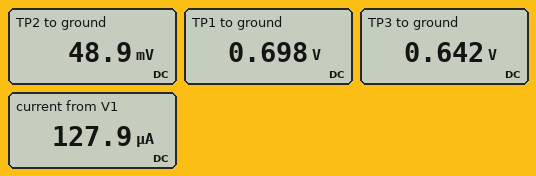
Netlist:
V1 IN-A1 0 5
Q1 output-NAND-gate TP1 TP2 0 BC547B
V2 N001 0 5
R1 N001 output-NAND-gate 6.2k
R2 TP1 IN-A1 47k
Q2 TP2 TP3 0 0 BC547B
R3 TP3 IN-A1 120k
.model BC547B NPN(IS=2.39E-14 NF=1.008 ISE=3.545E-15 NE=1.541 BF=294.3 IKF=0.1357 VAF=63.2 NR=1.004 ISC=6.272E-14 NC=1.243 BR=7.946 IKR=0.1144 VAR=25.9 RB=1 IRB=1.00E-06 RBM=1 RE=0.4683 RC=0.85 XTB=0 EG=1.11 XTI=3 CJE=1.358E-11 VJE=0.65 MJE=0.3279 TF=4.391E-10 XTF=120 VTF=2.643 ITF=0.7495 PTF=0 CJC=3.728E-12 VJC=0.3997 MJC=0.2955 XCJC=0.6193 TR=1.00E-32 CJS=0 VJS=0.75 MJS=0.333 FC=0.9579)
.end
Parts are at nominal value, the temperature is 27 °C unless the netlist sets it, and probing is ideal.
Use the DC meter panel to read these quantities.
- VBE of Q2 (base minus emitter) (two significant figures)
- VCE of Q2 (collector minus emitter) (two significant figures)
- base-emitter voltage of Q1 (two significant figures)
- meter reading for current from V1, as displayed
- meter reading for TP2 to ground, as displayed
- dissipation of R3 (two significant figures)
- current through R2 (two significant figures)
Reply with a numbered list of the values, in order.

1. 640 mV
2. 49 mV
3. 650 mV
4. 127.9 µA
5. 48.9 mV
6. 160 µW
7. 92 µA
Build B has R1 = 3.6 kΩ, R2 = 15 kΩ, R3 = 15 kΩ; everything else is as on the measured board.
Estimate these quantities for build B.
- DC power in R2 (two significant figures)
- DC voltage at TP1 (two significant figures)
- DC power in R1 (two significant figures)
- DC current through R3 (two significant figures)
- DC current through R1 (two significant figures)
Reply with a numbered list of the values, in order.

1. 1.2 mW
2. 700 mV
3. 6.8 mW
4. 290 µA
5. 1.4 mA
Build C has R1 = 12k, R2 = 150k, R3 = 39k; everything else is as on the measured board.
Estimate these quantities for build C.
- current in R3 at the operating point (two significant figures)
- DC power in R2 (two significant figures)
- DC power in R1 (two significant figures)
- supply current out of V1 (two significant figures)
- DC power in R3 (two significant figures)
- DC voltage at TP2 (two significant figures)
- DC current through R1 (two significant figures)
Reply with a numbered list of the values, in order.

1. 110 µA
2. 130 µW
3. 2.0 mW
4. 140 µA
5. 490 µW
6. 19 mV
7. 410 µA
